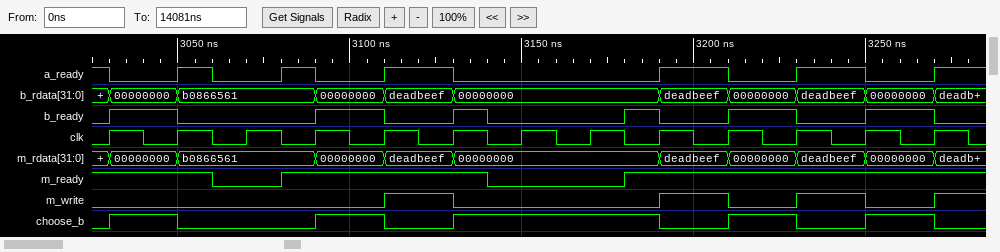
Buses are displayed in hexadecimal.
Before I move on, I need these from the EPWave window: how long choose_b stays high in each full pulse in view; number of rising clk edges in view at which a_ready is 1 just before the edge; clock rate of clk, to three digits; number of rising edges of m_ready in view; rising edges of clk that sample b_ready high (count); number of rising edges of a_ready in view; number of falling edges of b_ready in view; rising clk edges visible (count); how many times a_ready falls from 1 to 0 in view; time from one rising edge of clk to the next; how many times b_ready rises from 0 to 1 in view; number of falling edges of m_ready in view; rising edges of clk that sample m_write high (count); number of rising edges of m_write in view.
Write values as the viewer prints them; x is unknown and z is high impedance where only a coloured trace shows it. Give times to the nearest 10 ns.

20 ns, 20 ns, 60 ns, 20 ns, 20 ns
5
50.0 MHz
2
5
6
6
13
6
20 ns
6
2
3
4
